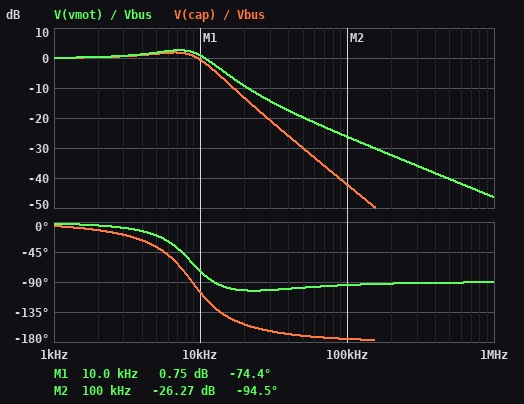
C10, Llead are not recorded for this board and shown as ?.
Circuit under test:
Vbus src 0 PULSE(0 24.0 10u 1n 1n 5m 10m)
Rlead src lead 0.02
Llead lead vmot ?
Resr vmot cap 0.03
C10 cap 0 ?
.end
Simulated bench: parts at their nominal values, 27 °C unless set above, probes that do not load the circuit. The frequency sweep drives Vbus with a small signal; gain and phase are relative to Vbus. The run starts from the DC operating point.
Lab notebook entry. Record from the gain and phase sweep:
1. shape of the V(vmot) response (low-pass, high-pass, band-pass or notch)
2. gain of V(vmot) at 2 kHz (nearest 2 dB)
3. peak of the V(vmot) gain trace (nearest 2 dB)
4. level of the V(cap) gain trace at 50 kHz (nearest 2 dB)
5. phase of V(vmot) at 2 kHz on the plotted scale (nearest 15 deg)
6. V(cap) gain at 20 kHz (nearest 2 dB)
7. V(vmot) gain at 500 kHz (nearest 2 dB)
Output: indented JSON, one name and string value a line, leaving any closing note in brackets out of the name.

{
  "shape of the V(vmot) response": "low-pass",
  "gain of V(vmot) at 2 kHz": "0 dB",
  "peak of the V(vmot) gain trace": "2 dB",
  "level of the V(cap) gain trace at 50 kHz": "-30 dB",
  "phase of V(vmot) at 2 kHz on the plotted scale": "0 deg",
  "V(cap) gain at 20 kHz": "-14 dB",
  "V(vmot) gain at 500 kHz": "-40 dB"
}
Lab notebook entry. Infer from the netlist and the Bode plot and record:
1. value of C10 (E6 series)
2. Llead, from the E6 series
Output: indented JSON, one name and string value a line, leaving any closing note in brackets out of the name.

{
  "value of C10": "330 µF",
  "Llead, from the E6 series": "1 µH"
}
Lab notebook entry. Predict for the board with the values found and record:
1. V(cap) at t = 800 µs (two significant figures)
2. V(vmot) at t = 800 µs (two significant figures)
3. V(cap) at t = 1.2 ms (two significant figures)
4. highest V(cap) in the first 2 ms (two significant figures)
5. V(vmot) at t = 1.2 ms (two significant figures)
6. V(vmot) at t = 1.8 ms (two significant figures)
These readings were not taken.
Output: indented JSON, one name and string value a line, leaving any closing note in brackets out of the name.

{
  "V(cap) at t = 800 µs": "24 V",
  "V(vmot) at t = 800 µs": "24 V",
  "V(cap) at t = 1.2 ms": "24 V",
  "highest V(cap) in the first 2 ms": "29 V",
  "V(vmot) at t = 1.2 ms": "24 V",
  "V(vmot) at t = 1.8 ms": "24 V"
}
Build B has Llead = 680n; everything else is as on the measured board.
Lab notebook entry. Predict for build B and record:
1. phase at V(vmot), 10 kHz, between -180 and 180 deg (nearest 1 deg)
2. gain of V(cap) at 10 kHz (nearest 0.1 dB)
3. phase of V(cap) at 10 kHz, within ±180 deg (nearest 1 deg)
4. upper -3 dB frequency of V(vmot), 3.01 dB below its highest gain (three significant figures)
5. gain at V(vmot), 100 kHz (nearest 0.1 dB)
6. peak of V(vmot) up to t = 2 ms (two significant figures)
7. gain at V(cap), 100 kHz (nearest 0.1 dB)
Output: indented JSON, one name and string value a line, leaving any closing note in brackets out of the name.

{
  "phase at V(vmot), 10 kHz, between -180 and 180 deg": "-52 deg",
  "gain of V(cap) at 10 kHz": "-0.4 dB",
  "phase of V(cap) at 10 kHz, within ±180 deg": "-84 deg",
  "upper -3 dB frequency of V(vmot), 3.01 dB below its highest gain": "13.6 kHz",
  "gain at V(vmot), 100 kHz": "-22.9 dB",
  "peak of V(vmot) up to t = 2 ms": "28 V",
  "gain at V(cap), 100 kHz": "-38.9 dB"
}
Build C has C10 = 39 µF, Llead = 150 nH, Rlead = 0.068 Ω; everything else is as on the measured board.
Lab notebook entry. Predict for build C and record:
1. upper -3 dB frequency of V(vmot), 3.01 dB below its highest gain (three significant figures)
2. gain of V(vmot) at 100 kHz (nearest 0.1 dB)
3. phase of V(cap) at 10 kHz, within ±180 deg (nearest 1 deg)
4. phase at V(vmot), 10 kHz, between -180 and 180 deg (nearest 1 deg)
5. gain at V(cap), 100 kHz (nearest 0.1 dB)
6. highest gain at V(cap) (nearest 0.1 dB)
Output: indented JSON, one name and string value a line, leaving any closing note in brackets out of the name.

{
  "upper -3 dB frequency of V(vmot), 3.01 dB below its highest gain": "65.3 kHz",
  "gain of V(vmot) at 100 kHz": "-6.9 dB",
  "phase of V(cap) at 10 kHz, within ±180 deg": "-14 deg",
  "phase at V(vmot), 10 kHz, between -180 and 180 deg": "-10 deg",
  "gain at V(cap), 100 kHz": "-8.7 dB",
  "highest gain at V(cap)": "0 dB"
}
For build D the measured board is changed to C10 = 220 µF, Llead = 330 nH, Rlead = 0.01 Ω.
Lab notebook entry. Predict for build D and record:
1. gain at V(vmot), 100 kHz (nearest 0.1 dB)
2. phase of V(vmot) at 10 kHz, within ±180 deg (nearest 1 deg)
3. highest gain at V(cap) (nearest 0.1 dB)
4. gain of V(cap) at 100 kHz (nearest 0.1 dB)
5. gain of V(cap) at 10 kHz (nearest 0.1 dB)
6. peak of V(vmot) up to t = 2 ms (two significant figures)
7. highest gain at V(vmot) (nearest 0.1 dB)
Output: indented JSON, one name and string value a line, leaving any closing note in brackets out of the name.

{
  "gain at V(vmot), 100 kHz": "-16.4 dB",
  "phase of V(vmot) at 10 kHz, within ±180 deg": "-15 deg",
  "highest gain at V(cap)": "1.1 dB",
  "gain of V(cap) at 100 kHz": "-29.0 dB",
  "gain of V(cap) at 10 kHz": "0.9 dB",
  "peak of V(vmot) up to t = 2 ms": "29 V",
  "highest gain at V(vmot)": "2.3 dB"
}
